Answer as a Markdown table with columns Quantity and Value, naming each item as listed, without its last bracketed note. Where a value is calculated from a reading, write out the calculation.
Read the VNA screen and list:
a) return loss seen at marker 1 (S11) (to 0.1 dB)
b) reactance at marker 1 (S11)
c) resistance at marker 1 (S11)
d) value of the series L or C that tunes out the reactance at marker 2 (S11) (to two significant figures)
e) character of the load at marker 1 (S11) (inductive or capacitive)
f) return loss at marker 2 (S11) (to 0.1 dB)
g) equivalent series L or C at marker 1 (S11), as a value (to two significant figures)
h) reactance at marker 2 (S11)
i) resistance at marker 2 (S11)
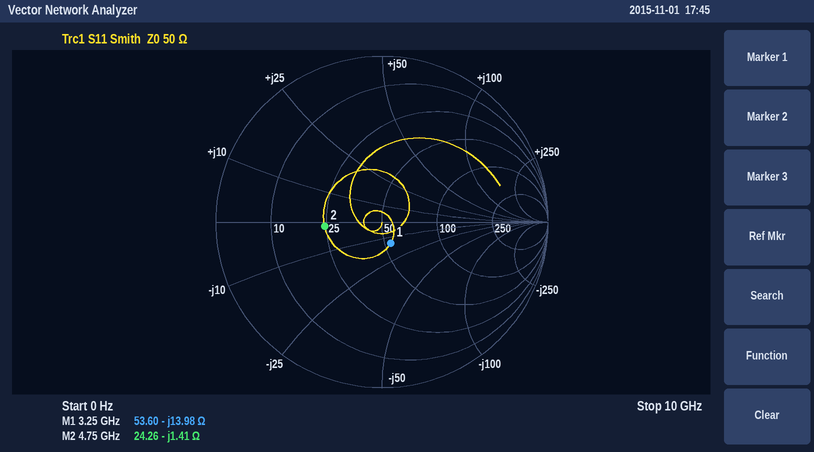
| Quantity | Value |
|---|---|
| return loss seen at marker 1 (S11) | 17.2 dB |
| reactance at marker 1 | -13.98 Ω |
| resistance at marker 1 | 53.60 Ω |
| value of the series L or C that tunes out the reactance at marker 2 (S11) | L = 1.41 Ω/(2π × 4.75 GHz) ≈ 47 pH |
| character of the load at marker 1 (S11) | capacitive |
| return loss at marker 2 (S11) | 9.2 dB |
| equivalent series L or C at marker 1 (S11), as a value | C = 1/(2π × 3.25 GHz × 13.98 Ω) ≈ 3.5 pF |
| reactance at marker 2 | -1.41 Ω |
| resistance at marker 2 | 24.26 Ω |
